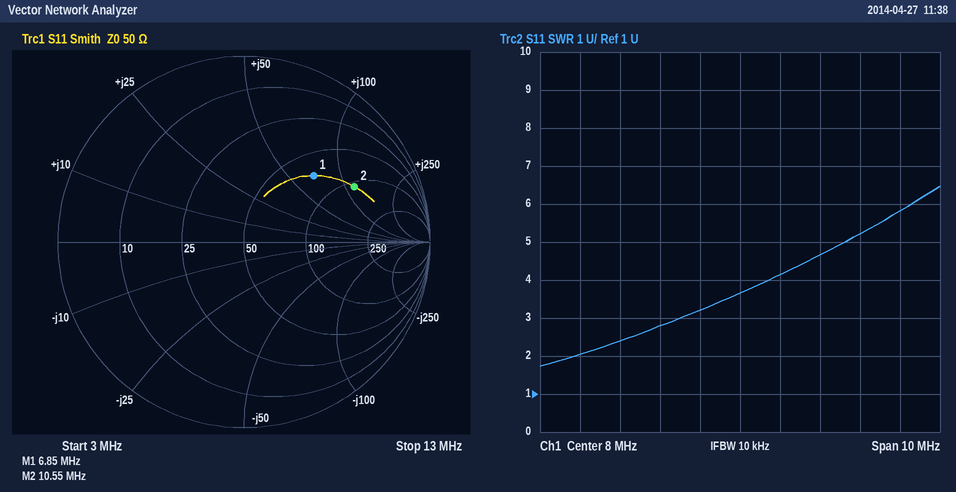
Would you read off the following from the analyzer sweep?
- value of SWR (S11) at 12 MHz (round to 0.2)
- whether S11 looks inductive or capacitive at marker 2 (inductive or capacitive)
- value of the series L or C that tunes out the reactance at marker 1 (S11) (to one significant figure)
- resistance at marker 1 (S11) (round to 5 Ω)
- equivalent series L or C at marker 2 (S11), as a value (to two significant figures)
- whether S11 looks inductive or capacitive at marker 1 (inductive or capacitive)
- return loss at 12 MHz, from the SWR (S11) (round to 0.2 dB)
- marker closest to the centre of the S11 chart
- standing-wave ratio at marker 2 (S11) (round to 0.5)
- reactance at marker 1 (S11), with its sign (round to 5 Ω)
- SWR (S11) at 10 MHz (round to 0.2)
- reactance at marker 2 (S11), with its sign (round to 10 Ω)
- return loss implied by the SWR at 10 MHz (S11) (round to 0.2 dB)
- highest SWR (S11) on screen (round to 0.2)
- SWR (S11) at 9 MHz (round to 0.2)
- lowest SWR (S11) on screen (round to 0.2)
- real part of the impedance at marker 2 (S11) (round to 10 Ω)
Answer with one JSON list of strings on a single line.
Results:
["5.8", "inductive", "300 pF", "70 Ω", "1.8 µH", "inductive", "3.0 dB", "marker 1", "5.0", "+70 Ω", "4.6", "+120 Ω", "3.8 dB", "6.4", "4.2", "1.8", "110 Ω"]
